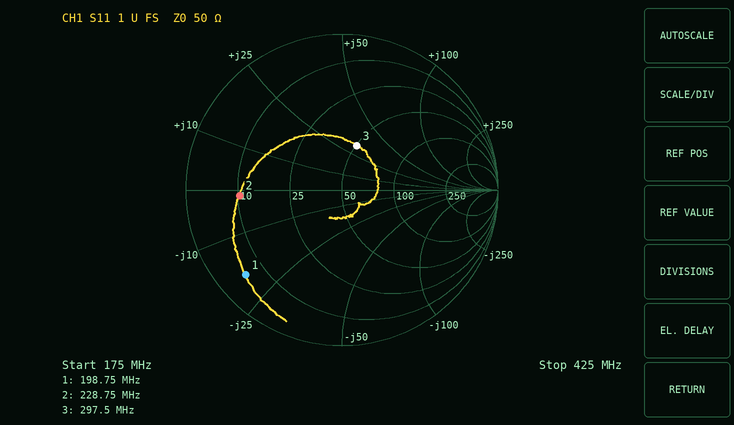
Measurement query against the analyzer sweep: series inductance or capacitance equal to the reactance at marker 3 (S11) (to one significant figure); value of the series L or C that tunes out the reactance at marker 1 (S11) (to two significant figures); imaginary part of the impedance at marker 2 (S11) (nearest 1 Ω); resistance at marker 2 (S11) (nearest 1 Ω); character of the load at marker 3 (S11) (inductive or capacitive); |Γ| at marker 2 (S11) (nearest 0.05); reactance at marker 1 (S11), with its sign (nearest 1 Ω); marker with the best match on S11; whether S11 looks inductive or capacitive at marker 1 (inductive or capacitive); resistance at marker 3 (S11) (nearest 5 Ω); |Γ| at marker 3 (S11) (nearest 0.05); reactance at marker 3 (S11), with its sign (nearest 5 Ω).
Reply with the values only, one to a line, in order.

20 nH
15 nH
-1 Ω
10 Ω
inductive
0.65
-19 Ω
marker 3
capacitive
50 Ω
0.30
+30 Ω
